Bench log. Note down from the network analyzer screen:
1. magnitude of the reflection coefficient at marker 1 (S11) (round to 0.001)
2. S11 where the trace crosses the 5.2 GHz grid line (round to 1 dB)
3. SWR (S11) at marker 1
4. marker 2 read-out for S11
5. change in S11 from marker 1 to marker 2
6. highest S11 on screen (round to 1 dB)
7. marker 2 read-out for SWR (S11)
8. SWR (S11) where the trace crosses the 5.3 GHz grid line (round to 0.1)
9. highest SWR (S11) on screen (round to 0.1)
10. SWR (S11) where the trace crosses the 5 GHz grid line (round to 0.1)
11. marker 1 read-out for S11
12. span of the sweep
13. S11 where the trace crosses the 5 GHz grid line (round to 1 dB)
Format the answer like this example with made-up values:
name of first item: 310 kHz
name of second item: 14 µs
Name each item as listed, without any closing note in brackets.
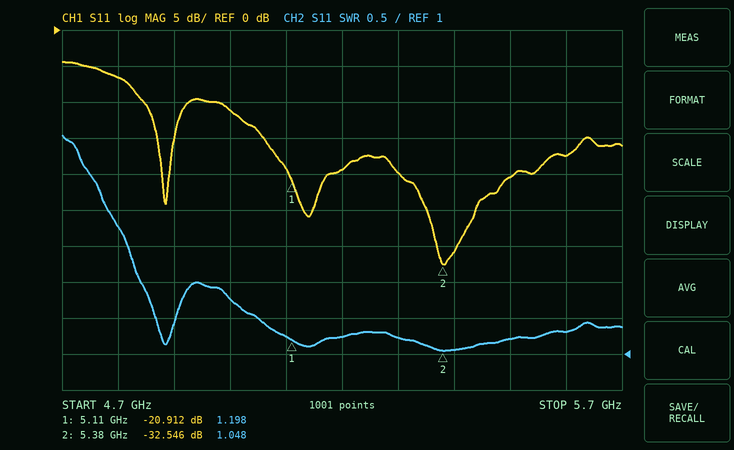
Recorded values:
magnitude of the reflection coefficient at marker 1 (S11): 0.090
S11 where the trace crosses the 5.2 GHz grid line: -19 dB
SWR (S11) at marker 1: 1.198
marker 2 read-out for S11: -32.546 dB
change in S11 from marker 1 to marker 2: -11.634 dB
highest S11 on screen: -4 dB
marker 2 read-out for SWR: 1.048
SWR (S11) where the trace crosses the 5.3 GHz grid line: 1.2
highest SWR (S11) on screen: 4.0
SWR (S11) where the trace crosses the 5 GHz grid line: 1.8
marker 1 read-out for S11: -20.912 dB
span of the sweep: 1 GHz
S11 where the trace crosses the 5 GHz grid line: -11 dB
